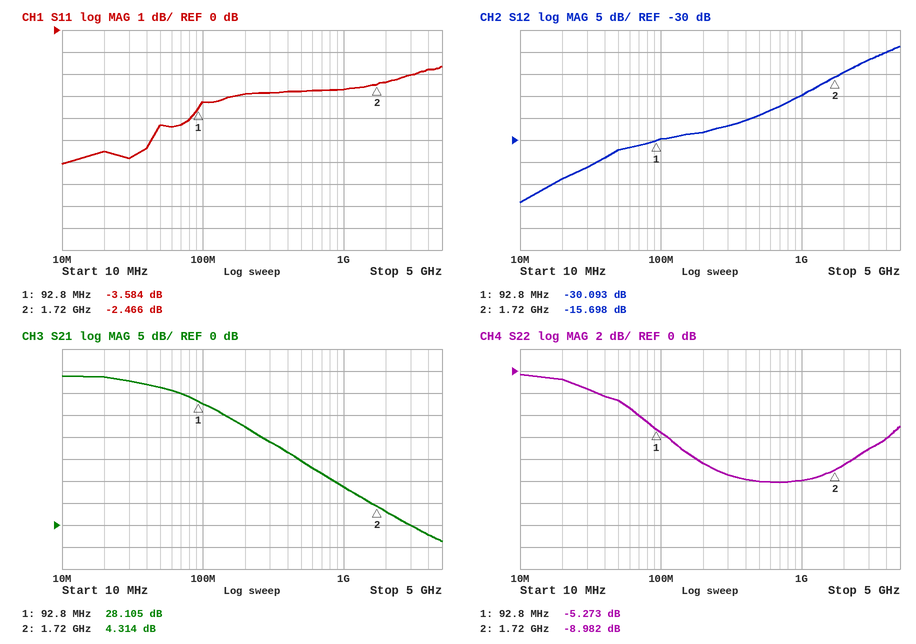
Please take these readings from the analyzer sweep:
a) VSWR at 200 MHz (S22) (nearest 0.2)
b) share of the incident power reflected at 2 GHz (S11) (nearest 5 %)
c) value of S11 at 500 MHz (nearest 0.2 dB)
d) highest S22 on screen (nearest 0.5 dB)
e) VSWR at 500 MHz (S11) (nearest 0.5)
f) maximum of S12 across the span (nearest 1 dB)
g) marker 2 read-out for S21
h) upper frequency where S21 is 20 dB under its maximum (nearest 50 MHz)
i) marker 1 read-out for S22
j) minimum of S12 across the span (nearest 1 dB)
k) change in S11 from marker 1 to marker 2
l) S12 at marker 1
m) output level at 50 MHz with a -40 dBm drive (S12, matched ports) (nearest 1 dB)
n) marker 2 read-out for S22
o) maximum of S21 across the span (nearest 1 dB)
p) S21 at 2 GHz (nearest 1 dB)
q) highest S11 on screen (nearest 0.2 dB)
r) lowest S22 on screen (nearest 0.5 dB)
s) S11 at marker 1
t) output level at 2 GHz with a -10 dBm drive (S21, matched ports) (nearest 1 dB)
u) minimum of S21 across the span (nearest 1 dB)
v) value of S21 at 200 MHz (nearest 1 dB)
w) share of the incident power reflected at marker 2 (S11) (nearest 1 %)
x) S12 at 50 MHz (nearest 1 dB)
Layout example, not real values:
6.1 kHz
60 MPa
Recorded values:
2.2
60 %
-2.8 dB
-0.5 dB
6.5
-9 dB
4.314 dB
550 MHz
-5.273 dB
-44 dB
1.118 dB
-30.093 dB
-72 dBm
-8.982 dB
34 dB
3 dB
-1.6 dB
-10.0 dB
-3.584 dB
-7 dBm
-4 dB
22 dB
57 %
-32 dB
